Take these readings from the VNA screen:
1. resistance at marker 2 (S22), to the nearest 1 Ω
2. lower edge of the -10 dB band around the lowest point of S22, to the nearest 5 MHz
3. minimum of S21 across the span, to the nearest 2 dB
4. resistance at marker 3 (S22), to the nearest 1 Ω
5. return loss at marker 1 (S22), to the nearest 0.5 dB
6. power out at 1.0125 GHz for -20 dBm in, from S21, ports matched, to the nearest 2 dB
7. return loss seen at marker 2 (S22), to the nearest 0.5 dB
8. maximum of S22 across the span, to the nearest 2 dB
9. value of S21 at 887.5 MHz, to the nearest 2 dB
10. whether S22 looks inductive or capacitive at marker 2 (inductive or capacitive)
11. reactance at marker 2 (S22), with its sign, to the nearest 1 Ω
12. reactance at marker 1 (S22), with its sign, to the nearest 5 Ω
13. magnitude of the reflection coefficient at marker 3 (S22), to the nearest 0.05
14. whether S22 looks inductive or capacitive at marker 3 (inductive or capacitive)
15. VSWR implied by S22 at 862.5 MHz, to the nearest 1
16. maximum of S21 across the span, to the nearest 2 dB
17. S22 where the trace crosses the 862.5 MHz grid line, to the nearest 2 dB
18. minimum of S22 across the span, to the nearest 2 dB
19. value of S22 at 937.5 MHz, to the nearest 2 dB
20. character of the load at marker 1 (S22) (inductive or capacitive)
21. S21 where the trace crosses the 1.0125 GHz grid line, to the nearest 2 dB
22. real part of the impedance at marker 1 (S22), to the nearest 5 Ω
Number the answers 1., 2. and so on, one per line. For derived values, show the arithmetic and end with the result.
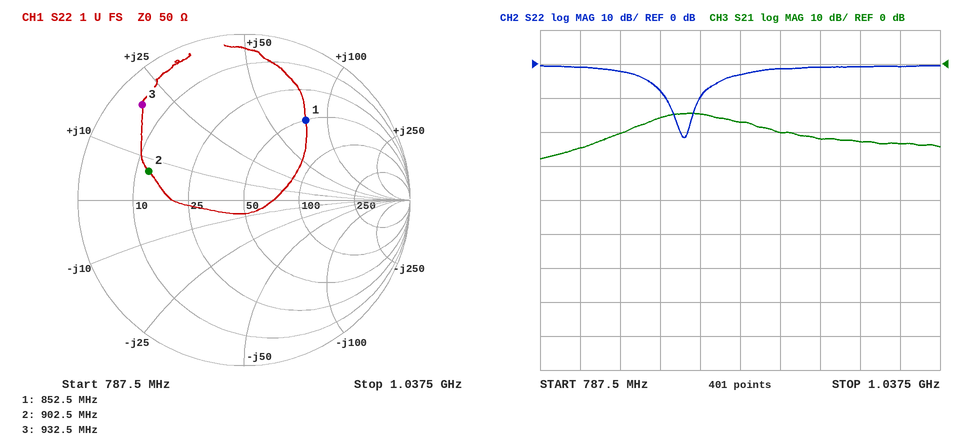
1. 13 Ω
2. 865 MHz
3. -28 dB
4. 5 Ω
5. 4.5 dB
6. -20 dBm + (-24 dB) = -44 dBm
7. 4.5 dB
8. 0 dB
9. -14 dB
10. inductive
11. +7 Ω
12. +75 Ω
13. 0.85
14. inductive
15. |Γ| = 10^(-8/20) = 0.3981; VSWR = (1 + 0.3981)/(1 − 0.3981) ≈ 2
16. -14 dB
17. -8 dB
18. -22 dB
19. -2 dB
20. inductive
21. -24 dB
22. 50 Ω
